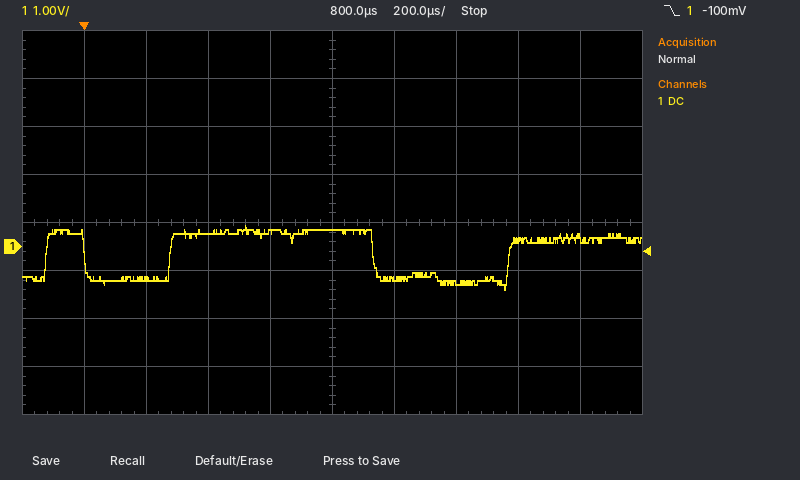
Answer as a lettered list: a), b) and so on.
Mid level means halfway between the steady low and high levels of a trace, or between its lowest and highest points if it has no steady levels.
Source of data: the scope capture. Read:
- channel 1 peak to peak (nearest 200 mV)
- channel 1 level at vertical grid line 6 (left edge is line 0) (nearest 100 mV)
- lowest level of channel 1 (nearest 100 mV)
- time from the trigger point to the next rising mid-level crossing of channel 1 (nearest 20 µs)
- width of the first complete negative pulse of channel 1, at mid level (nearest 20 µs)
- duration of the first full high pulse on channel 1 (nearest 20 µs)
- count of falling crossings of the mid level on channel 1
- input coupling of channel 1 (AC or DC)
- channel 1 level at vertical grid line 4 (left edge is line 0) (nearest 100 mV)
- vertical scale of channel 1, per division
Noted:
a) 1.4 V
b) -700 mV
c) -900 mV
d) 280 µs
e) 280 µs
f) 120 µs
g) 2
h) DC
i) 300 mV
j) 1 V
